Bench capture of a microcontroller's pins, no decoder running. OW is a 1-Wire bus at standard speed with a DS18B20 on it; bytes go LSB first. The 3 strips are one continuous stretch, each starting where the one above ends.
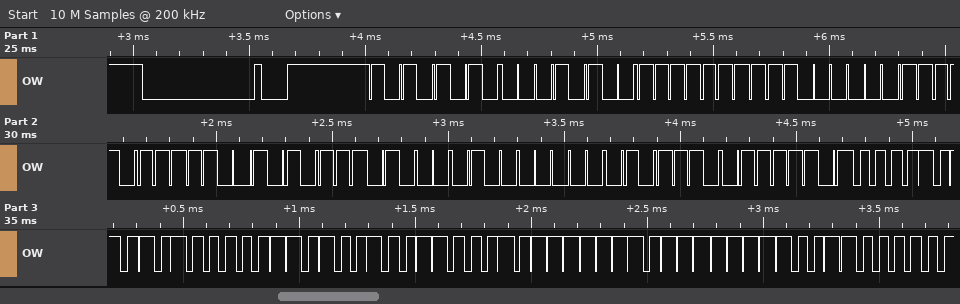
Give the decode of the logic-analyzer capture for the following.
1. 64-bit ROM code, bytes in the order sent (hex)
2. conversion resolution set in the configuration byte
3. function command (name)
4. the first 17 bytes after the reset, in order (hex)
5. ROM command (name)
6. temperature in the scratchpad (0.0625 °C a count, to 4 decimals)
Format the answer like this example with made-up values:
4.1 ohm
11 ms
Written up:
28 FF 03 EF 53 17 02 74
12 bits
Read Scratchpad
55 28 FF 03 EF 53 17 02 74 BE 50 05 4B 46 7F FF 0C
Match ROM
85.0000 °C
